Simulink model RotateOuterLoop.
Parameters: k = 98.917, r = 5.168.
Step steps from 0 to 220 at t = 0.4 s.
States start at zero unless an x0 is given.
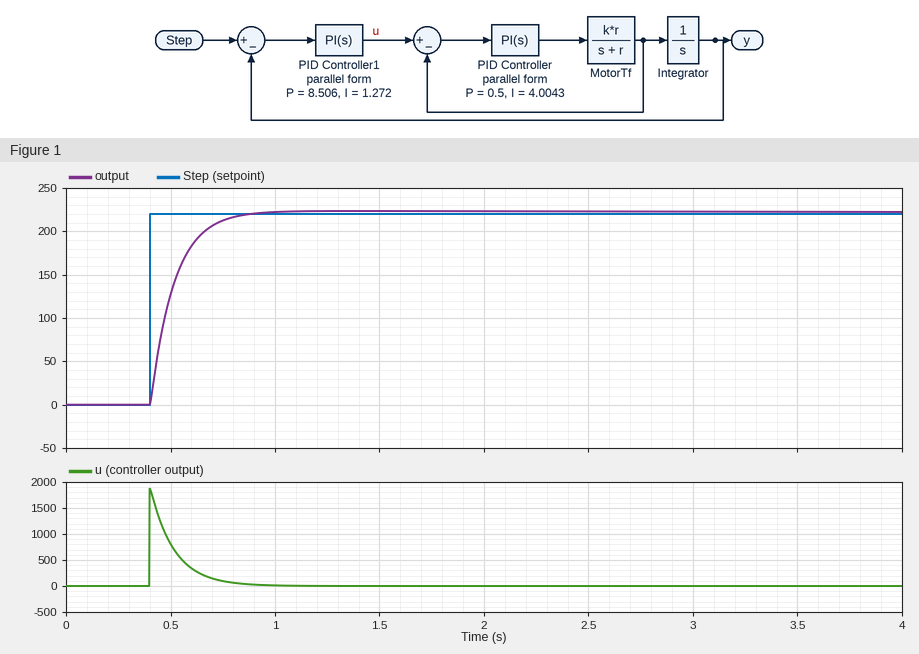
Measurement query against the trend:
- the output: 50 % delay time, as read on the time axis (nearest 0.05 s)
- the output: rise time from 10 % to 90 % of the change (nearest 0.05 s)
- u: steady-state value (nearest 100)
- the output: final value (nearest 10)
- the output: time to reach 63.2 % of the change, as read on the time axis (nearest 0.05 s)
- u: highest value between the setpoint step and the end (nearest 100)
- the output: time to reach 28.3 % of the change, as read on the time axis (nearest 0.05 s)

0.50 s
0.25 s
0
220
0.50 s
1900
0.45 s
